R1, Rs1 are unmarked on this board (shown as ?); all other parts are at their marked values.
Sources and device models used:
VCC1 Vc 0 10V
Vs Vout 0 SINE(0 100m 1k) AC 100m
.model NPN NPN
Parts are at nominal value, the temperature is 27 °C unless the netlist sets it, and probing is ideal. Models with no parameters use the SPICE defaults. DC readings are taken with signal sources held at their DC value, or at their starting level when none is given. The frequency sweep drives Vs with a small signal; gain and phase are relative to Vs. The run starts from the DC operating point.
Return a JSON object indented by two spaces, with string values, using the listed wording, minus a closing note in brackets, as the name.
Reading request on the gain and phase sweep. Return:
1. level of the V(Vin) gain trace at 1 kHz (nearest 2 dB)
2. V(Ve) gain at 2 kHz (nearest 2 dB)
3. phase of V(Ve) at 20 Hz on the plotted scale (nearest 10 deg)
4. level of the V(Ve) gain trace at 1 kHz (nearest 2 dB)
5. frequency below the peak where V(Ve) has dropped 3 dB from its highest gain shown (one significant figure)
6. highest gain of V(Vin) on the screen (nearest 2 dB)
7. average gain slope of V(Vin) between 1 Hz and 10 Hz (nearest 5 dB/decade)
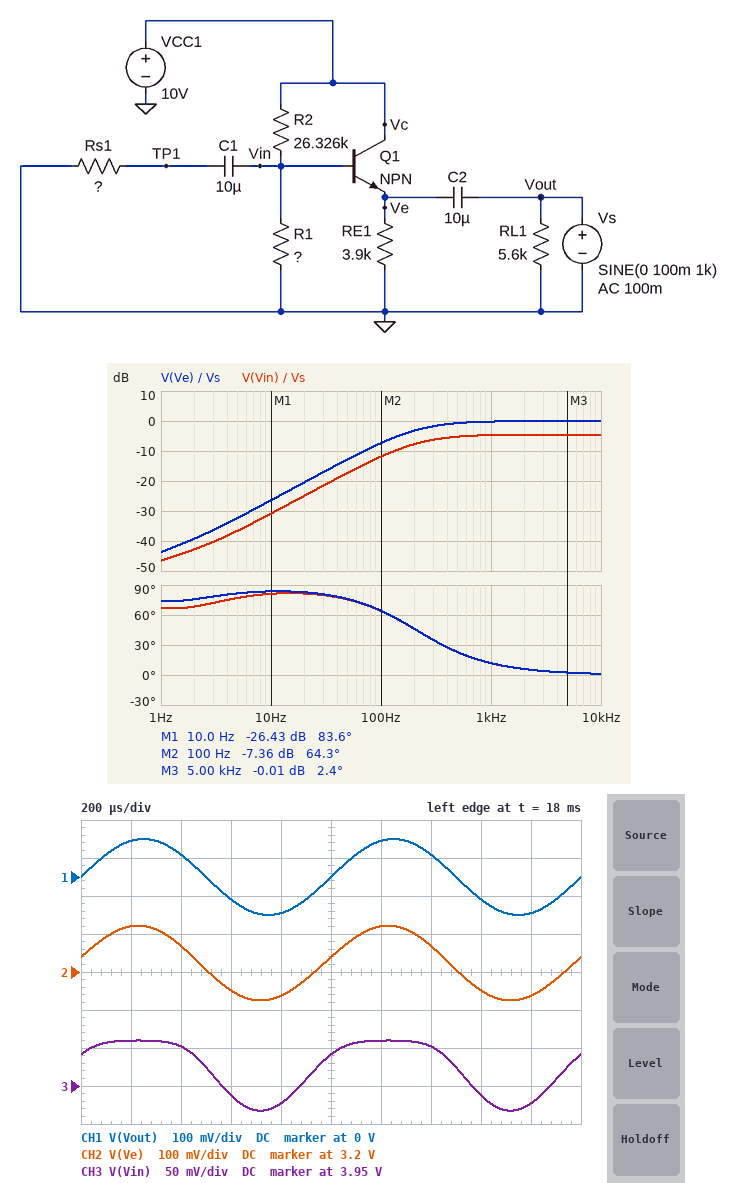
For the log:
{
  "level of the V(Vin) gain trace at 1 kHz": "-4 dB",
  "V(Ve) gain at 2 kHz": "0 dB",
  "phase of V(Ve) at 20 Hz on the plotted scale": "80 deg",
  "level of the V(Ve) gain trace at 1 kHz": "0 dB",
  "frequency below the peak where V(Ve) has dropped 3 dB from its highest gain shown": "200 Hz",
  "highest gain of V(Vin) on the screen": "-4 dB",
  "average gain slope of V(Vin) between 1 Hz and 10 Hz": "15 dB/decade"
}
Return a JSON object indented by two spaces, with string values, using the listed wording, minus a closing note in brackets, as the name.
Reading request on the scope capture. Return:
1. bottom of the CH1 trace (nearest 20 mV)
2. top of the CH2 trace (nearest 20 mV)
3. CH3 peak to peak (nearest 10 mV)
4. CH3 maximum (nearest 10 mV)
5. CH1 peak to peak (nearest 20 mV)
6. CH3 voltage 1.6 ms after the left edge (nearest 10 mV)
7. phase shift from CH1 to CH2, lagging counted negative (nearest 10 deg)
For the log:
{
  "bottom of the CH1 trace": "-100 mV",
  "top of the CH2 trace": "3.32 V",
  "CH3 peak to peak": "90 mV",
  "CH3 maximum": "4.01 V",
  "CH1 peak to peak": "200 mV",
  "CH3 voltage 1.6 ms after the left edge": "3.94 V",
  "phase shift from CH1 to CH2, lagging counted negative": "10 deg"
}
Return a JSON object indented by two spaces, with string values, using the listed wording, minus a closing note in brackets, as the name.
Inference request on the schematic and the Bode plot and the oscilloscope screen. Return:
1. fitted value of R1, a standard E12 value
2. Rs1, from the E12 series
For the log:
{
  "fitted value of R1, a standard E12 value": "18 kΩ",
  "Rs1, from the E12 series": "8.2 kΩ"
}
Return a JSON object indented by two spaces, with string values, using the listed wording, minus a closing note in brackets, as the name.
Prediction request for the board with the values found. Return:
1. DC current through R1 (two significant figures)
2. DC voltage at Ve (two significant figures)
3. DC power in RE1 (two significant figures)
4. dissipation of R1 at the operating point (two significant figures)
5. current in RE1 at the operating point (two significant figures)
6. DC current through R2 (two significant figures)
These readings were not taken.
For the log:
{
  "DC current through R1": "220 µA",
  "DC voltage at Ve": "3.2 V",
  "DC power in RE1": "2.6 mW",
  "dissipation of R1 at the operating point": "880 µW",
  "current in RE1 at the operating point": "820 µA",
  "DC current through R2": "230 µA"
}
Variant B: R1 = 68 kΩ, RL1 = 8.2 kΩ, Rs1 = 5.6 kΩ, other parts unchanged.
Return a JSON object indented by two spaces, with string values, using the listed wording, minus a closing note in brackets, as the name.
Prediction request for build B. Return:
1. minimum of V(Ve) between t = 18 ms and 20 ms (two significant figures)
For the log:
{
  "minimum of V(Ve) between t = 18 ms and 20 ms": "6.0 V"
}
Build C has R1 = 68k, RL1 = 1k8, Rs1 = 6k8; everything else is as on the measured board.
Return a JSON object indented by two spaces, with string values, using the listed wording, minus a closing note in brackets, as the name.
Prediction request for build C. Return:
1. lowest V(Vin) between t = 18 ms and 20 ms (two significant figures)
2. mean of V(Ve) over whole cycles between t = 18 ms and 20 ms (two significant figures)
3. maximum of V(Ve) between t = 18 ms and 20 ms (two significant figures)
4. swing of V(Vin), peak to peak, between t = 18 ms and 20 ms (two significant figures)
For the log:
{
  "lowest V(Vin) between t = 18 ms and 20 ms": "6.8 V",
  "mean of V(Ve) over whole cycles between t = 18 ms and 20 ms": "6.1 V",
  "maximum of V(Ve) between t = 18 ms and 20 ms": "6.2 V",
  "swing of V(Vin), peak to peak, between t = 18 ms and 20 ms": "140 mV"
}
